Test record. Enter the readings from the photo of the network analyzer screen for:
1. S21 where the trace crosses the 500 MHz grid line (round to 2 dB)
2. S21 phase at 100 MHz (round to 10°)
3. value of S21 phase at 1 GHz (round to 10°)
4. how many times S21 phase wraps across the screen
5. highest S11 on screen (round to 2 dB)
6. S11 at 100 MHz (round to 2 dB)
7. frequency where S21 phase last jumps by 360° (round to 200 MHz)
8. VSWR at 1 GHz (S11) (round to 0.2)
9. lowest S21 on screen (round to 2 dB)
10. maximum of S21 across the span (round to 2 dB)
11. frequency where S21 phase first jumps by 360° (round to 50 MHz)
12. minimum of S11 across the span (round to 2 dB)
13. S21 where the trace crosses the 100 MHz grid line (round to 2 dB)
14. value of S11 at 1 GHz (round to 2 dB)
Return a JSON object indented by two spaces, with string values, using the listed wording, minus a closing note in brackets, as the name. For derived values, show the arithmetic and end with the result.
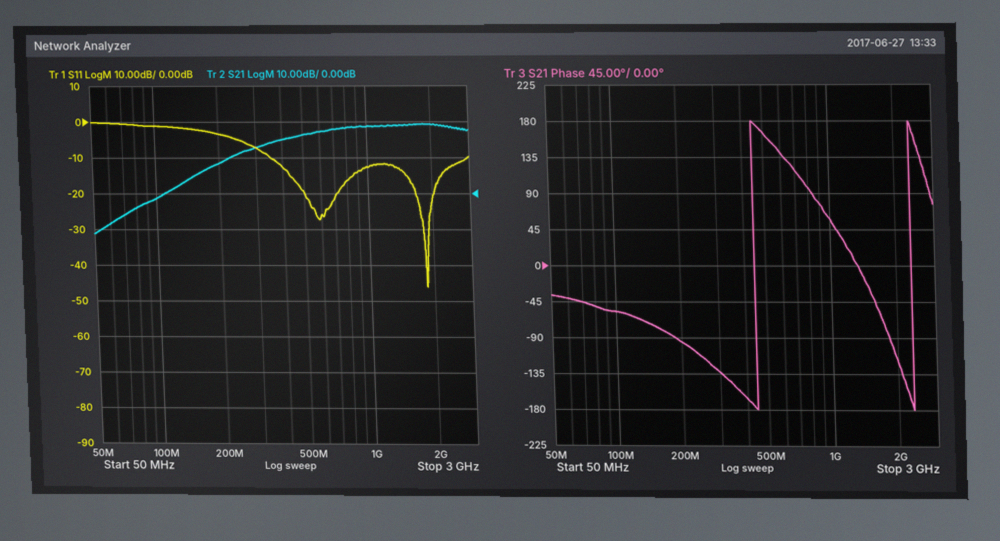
{
  "S21 where the trace crosses the 500 MHz grid line": "16 dB",
  "S21 phase at 100 MHz": "-60°",
  "value of S21 phase at 1 GHz": "60°",
  "how many times S21 phase wraps across the screen": "2",
  "highest S11 on screen": "0 dB",
  "S11 at 100 MHz": "-2 dB",
  "frequency where S21 phase last jumps by 360°": "2.4 GHz",
  "VSWR at 1 GHz (S11)": "|Γ| = 10^(-12/20) = 0.2512; VSWR = (1 + 0.2512)/(1 − 0.2512) ≈ 1.67, so 1.6 to the nearest 0.2",
  "lowest S21 on screen": "-12 dB",
  "maximum of S21 across the span": "20 dB",
  "frequency where S21 phase first jumps by 360°": "450 MHz",
  "minimum of S11 across the span": "-46 dB",
  "S21 where the trace crosses the 100 MHz grid line": "-2 dB",
  "value of S11 at 1 GHz": "-12 dB"
}
